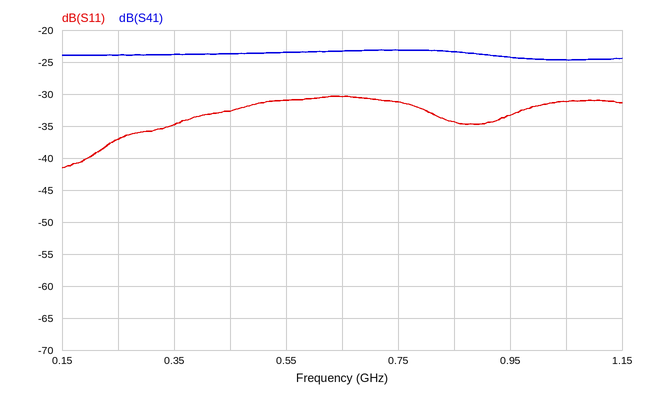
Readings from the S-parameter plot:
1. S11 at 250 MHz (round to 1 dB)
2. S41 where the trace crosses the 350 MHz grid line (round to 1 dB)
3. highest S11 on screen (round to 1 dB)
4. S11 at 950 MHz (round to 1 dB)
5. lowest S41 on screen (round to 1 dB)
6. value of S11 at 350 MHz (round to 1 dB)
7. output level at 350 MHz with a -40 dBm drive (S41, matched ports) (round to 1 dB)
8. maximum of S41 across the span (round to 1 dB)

-37 dB
-24 dB
-30 dB
-33 dB
-25 dB
-35 dB
-64 dBm
-23 dB
